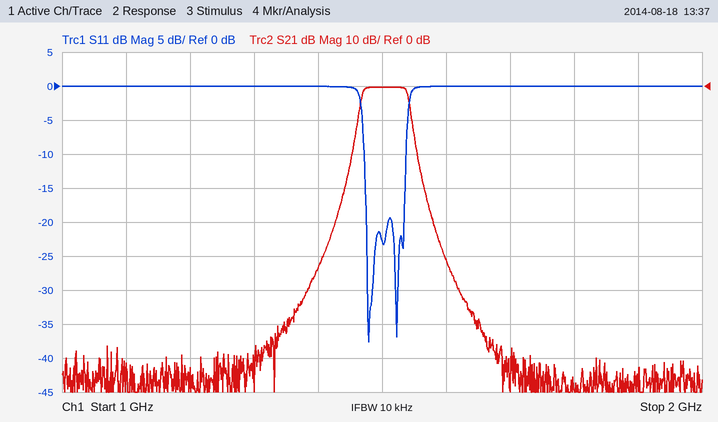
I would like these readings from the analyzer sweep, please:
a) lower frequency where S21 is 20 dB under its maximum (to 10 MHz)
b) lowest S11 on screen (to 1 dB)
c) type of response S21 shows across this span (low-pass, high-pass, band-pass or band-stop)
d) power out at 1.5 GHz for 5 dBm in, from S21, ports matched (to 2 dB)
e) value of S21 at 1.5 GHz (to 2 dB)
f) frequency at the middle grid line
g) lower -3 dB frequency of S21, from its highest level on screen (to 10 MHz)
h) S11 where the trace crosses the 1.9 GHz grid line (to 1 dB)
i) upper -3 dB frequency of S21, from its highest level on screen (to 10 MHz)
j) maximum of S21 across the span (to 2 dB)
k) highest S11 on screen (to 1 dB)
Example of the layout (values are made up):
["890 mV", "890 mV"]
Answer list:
["1.45 GHz", "-38 dB", "band-pass", "4 dBm", "0 dB", "1.5 GHz", "1.47 GHz", "0 dB", "1.54 GHz", "0 dB", "0 dB"]
